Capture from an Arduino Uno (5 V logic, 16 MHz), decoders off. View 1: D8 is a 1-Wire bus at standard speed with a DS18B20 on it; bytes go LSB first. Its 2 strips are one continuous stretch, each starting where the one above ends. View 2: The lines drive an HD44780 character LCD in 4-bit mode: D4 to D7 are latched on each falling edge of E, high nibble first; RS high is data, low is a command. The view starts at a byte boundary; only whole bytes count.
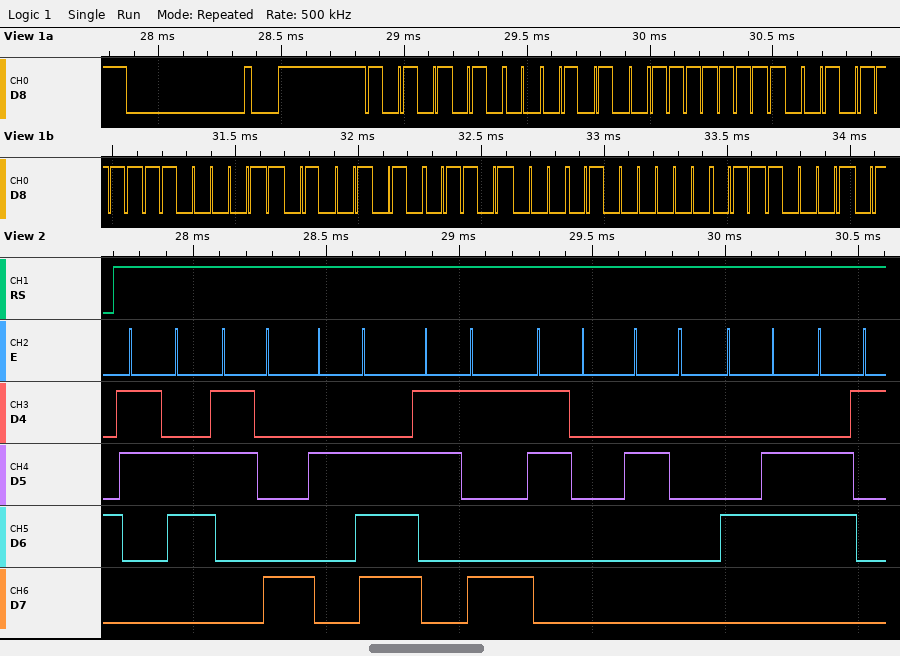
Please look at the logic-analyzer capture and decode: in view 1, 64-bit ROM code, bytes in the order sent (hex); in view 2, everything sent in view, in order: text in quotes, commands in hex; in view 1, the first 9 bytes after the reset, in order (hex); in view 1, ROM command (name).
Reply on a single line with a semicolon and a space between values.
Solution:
28 FF F4 C3 52 16 02 8E; "68.90 Fa"; 55 28 FF F4 C3 52 16 02 8E; Match ROM
